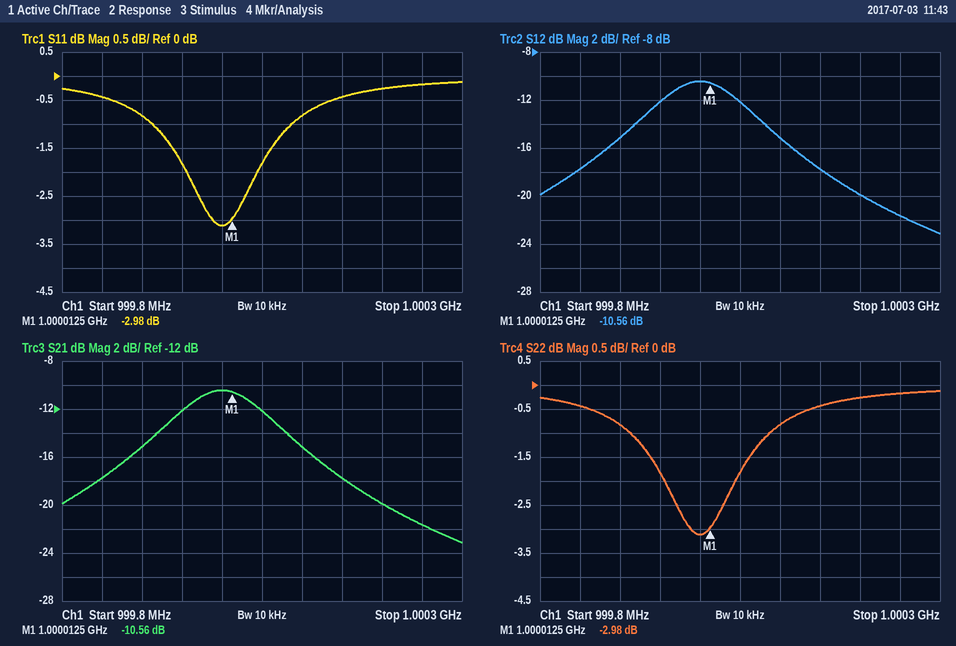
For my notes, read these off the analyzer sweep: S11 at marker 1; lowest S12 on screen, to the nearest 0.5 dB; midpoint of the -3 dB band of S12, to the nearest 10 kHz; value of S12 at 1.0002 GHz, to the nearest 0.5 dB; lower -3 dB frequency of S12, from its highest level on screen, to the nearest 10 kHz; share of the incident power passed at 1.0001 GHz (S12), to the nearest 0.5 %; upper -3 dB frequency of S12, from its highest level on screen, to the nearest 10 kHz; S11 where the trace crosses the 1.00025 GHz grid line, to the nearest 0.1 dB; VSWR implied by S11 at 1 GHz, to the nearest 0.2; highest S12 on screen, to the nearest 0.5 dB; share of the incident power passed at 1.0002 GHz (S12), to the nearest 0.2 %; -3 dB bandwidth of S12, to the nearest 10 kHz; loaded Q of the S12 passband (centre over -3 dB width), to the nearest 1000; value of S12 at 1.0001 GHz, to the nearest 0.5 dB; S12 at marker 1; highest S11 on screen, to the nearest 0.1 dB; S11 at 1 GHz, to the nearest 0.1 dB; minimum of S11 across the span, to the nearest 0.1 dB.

-2.98 dB
-23.0 dB
1.00000 GHz
-20.0 dB
999.93 MHz
3.0 %
1.00007 GHz
-0.2 dB
5.6
-10.5 dB
1.0 %
140 kHz
7000
-15.0 dB
-10.56 dB
-0.1 dB
-3.1 dB
-3.1 dB
